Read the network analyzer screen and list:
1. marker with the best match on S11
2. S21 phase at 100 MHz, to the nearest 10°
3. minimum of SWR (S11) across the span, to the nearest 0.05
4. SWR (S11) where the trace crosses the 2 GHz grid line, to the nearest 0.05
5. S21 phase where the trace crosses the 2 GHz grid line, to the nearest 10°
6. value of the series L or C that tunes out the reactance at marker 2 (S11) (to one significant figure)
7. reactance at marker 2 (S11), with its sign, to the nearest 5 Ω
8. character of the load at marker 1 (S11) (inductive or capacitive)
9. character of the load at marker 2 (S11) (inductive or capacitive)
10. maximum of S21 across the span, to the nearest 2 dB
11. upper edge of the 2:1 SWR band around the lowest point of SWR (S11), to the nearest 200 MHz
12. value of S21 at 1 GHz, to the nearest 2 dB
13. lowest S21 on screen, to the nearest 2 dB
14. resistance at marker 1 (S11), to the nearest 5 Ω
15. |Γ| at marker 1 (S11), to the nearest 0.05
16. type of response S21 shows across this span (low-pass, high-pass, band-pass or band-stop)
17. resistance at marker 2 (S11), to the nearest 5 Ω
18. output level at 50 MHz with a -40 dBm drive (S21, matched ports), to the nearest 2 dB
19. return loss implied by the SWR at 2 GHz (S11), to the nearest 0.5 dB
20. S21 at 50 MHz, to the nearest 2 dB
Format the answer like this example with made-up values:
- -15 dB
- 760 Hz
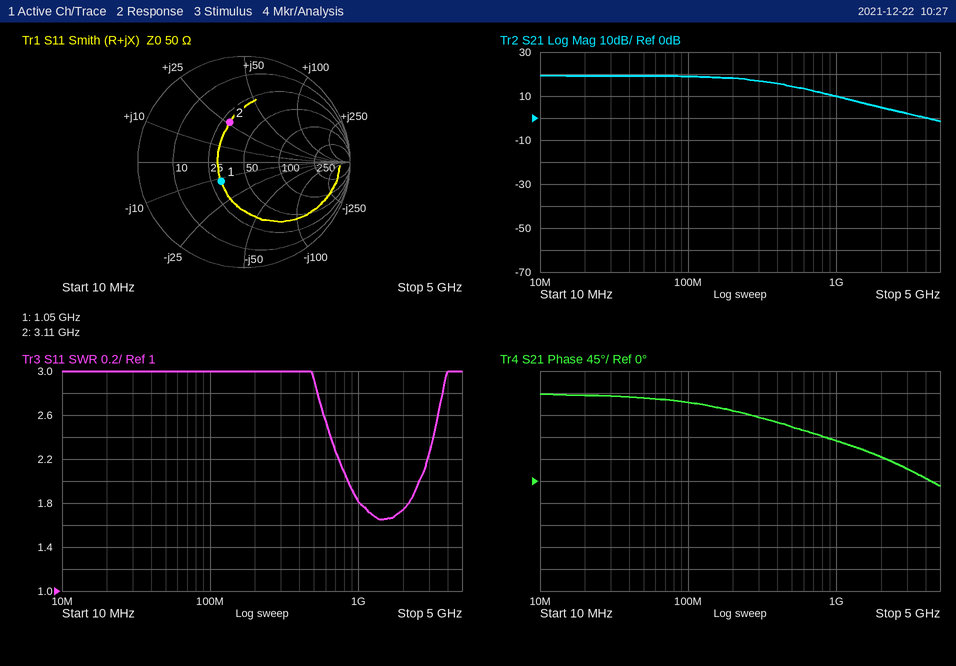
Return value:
- marker 1
- 160°
- 1.65
- 1.75
- 50°
- 2 pF
- +25 Ω
- capacitive
- inductive
- 20 dB
- 2.6 GHz
- 10 dB
- -2 dB
- 30 Ω
- 0.30
- low-pass
- 30 Ω
- -20 dBm
- 11.5 dB
- 20 dB
